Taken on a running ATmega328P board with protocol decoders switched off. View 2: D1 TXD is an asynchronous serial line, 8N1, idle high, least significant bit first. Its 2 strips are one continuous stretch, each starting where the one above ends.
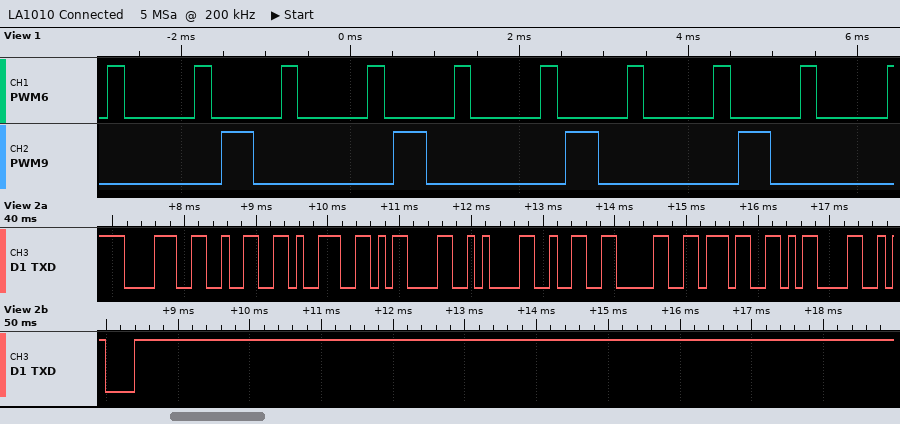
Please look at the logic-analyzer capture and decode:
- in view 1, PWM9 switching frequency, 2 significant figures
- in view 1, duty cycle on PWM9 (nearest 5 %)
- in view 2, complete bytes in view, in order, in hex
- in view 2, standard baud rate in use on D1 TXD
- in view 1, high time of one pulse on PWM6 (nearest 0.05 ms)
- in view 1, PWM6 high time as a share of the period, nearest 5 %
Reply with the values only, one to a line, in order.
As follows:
490 Hz
20 %
38 32 39 0D 0A 32 30 37 0D 0A
9600 baud
0.20 ms
20 %
